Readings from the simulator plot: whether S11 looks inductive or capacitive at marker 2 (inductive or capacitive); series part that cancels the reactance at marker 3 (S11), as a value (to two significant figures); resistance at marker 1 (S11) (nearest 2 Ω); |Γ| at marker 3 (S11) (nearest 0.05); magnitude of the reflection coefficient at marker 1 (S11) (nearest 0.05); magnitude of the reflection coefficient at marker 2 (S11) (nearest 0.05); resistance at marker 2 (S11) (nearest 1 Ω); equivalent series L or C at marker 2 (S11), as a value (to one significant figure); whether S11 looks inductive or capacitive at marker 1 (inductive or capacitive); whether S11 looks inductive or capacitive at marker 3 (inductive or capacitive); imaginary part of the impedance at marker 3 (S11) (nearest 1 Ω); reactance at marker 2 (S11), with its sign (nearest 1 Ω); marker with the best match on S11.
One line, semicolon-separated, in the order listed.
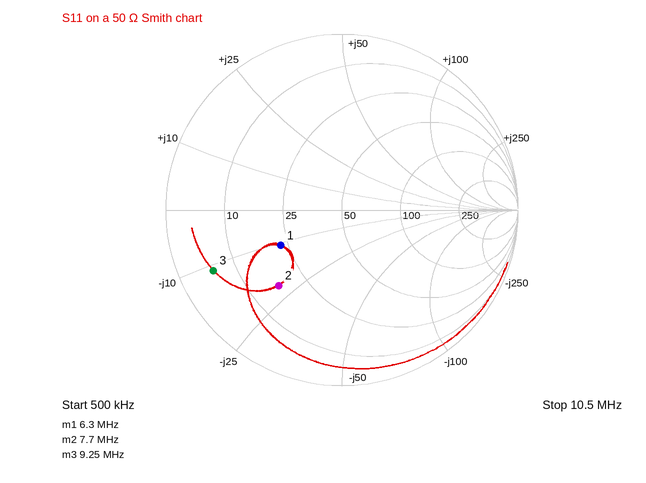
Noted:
capacitive; 190 nH; 22 Ω; 0.80; 0.40; 0.55; 17 Ω; 1.0 nF; capacitive; capacitive; -11 Ω; -21 Ω; marker 1
